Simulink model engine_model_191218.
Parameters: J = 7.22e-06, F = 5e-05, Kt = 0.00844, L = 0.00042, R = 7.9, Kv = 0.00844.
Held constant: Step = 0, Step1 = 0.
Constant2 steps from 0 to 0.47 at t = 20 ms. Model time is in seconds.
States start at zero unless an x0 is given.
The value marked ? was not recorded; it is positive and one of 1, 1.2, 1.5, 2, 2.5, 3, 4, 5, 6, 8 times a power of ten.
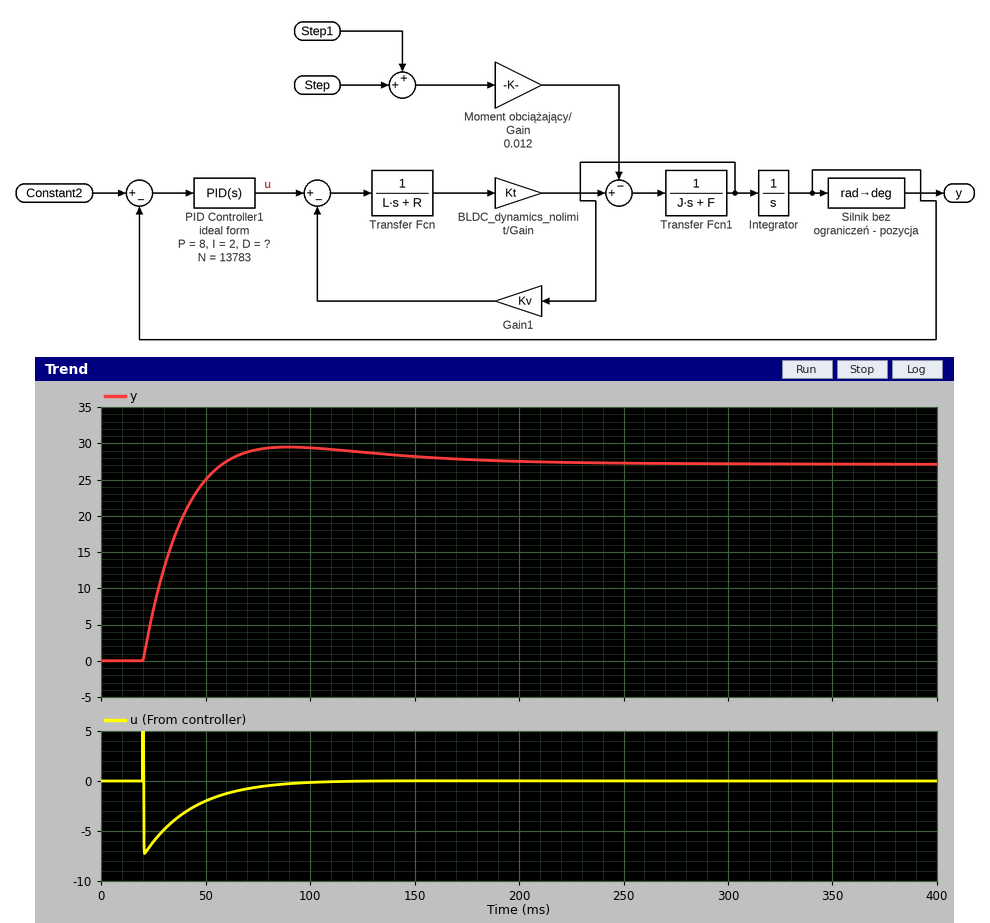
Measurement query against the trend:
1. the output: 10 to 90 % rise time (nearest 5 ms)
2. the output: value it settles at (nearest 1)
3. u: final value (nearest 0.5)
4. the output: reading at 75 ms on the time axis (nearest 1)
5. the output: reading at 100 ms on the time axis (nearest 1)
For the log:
25 ms
27
0.0
29
29
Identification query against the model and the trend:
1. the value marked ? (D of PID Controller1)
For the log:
0.05
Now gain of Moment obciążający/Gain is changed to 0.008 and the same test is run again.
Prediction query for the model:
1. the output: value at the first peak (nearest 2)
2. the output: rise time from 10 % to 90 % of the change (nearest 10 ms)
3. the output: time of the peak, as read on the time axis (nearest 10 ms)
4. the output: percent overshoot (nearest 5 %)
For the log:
30
30 ms
90 ms
10 %
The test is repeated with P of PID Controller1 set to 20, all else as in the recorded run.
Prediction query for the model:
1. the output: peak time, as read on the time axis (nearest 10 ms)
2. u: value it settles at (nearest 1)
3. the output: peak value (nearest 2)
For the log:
60 ms
0
28
